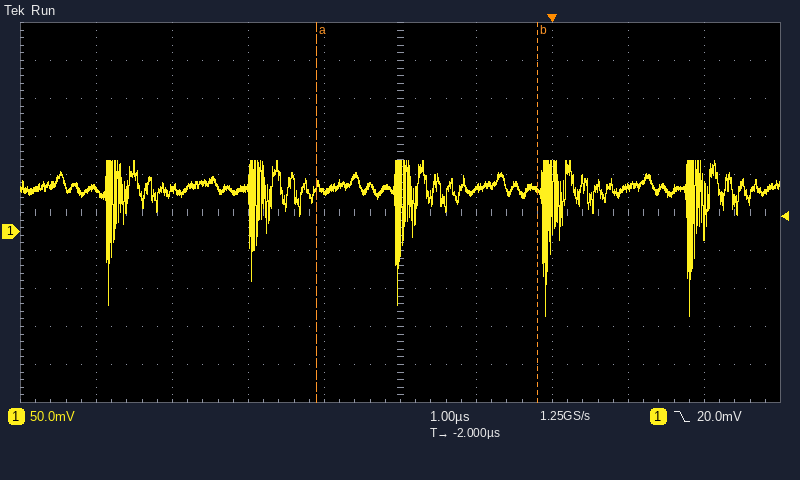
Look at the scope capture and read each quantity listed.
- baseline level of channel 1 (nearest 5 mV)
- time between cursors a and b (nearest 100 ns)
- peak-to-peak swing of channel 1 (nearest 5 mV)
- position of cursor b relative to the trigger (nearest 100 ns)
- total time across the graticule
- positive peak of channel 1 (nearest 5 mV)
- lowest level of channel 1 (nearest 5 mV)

55 mV
2.9 µs
205 mV
-200 ns
10 µs
95 mV
-110 mV
